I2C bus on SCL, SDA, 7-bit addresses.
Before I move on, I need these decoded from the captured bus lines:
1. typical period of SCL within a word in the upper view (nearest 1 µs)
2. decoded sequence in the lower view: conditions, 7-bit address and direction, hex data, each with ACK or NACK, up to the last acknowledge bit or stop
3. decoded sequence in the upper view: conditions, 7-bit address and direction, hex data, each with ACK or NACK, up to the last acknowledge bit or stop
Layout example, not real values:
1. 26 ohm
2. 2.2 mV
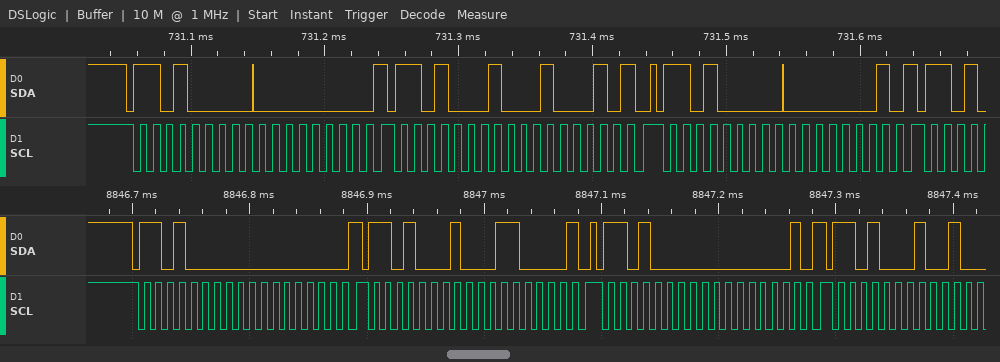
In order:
1. 10 µs
2. start, address 68 write ACK, 00 ACK, repeated start, address 68 read ACK, 30 NACK, stop, start, address 68 write ACK, 01 ACK, repeated start, address 68 read ACK
3. start, address 68 write ACK, 00 ACK, repeated start, address 68 read ACK, 22 NACK, stop, start, address 68 write ACK, 01 ACK
